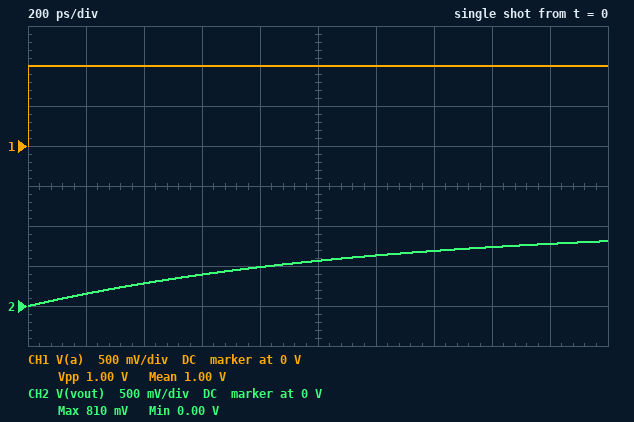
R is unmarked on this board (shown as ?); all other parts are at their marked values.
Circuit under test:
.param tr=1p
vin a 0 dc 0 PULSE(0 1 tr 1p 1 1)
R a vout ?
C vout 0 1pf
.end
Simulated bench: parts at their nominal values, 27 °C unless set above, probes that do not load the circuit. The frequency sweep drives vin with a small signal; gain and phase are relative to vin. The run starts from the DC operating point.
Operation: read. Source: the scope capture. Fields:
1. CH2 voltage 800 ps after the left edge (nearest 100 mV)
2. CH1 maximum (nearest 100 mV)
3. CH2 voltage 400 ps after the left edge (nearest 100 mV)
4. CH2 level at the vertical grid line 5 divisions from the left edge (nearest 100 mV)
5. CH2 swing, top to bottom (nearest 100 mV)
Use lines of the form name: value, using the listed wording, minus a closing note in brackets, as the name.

CH2 voltage 800 ps after the left edge: 500 mV
CH1 maximum: 1.0 V
CH2 voltage 400 ps after the left edge: 300 mV
CH2 level at the vertical grid line 5 divisions from the left edge: 600 mV
CH2 swing, top to bottom: 800 mV
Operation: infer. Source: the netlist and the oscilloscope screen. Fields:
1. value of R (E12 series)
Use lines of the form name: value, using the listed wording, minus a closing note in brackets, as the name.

value of R: 1.2 kΩ
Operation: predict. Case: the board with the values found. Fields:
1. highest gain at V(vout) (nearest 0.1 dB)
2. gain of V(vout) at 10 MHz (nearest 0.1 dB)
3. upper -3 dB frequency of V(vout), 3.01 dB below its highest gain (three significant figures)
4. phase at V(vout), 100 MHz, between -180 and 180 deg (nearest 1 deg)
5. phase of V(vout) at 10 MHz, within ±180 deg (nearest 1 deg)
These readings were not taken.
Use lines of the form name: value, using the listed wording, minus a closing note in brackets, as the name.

highest gain at V(vout): 0 dB
gain of V(vout) at 10 MHz: 0 dB
upper -3 dB frequency of V(vout), 3.01 dB below its highest gain: 133 MHz
phase at V(vout), 100 MHz, between -180 and 180 deg: -37 deg
phase of V(vout) at 10 MHz, within ±180 deg: -4 deg
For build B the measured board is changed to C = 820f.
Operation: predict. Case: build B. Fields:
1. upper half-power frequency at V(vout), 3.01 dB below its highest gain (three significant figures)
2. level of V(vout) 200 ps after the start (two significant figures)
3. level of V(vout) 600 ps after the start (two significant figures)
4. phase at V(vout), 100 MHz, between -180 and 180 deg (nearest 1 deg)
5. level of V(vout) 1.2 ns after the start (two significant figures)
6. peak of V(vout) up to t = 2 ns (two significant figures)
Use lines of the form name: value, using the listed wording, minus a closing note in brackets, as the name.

upper half-power frequency at V(vout), 3.01 dB below its highest gain: 162 MHz
level of V(vout) 200 ps after the start: 180 mV
level of V(vout) 600 ps after the start: 460 mV
phase at V(vout), 100 MHz, between -180 and 180 deg: -32 deg
level of V(vout) 1.2 ns after the start: 700 mV
peak of V(vout) up to t = 2 ns: 870 mV
